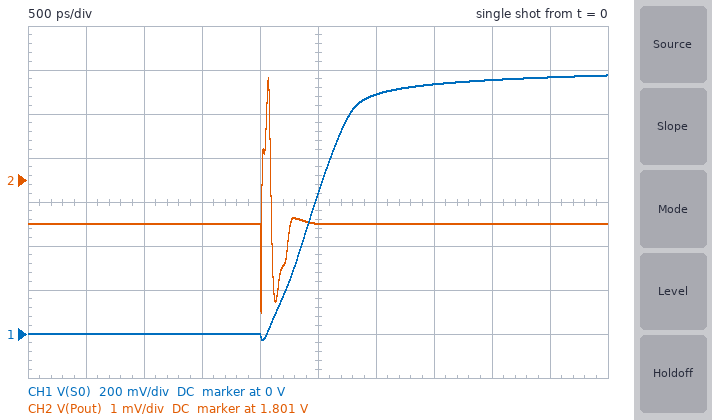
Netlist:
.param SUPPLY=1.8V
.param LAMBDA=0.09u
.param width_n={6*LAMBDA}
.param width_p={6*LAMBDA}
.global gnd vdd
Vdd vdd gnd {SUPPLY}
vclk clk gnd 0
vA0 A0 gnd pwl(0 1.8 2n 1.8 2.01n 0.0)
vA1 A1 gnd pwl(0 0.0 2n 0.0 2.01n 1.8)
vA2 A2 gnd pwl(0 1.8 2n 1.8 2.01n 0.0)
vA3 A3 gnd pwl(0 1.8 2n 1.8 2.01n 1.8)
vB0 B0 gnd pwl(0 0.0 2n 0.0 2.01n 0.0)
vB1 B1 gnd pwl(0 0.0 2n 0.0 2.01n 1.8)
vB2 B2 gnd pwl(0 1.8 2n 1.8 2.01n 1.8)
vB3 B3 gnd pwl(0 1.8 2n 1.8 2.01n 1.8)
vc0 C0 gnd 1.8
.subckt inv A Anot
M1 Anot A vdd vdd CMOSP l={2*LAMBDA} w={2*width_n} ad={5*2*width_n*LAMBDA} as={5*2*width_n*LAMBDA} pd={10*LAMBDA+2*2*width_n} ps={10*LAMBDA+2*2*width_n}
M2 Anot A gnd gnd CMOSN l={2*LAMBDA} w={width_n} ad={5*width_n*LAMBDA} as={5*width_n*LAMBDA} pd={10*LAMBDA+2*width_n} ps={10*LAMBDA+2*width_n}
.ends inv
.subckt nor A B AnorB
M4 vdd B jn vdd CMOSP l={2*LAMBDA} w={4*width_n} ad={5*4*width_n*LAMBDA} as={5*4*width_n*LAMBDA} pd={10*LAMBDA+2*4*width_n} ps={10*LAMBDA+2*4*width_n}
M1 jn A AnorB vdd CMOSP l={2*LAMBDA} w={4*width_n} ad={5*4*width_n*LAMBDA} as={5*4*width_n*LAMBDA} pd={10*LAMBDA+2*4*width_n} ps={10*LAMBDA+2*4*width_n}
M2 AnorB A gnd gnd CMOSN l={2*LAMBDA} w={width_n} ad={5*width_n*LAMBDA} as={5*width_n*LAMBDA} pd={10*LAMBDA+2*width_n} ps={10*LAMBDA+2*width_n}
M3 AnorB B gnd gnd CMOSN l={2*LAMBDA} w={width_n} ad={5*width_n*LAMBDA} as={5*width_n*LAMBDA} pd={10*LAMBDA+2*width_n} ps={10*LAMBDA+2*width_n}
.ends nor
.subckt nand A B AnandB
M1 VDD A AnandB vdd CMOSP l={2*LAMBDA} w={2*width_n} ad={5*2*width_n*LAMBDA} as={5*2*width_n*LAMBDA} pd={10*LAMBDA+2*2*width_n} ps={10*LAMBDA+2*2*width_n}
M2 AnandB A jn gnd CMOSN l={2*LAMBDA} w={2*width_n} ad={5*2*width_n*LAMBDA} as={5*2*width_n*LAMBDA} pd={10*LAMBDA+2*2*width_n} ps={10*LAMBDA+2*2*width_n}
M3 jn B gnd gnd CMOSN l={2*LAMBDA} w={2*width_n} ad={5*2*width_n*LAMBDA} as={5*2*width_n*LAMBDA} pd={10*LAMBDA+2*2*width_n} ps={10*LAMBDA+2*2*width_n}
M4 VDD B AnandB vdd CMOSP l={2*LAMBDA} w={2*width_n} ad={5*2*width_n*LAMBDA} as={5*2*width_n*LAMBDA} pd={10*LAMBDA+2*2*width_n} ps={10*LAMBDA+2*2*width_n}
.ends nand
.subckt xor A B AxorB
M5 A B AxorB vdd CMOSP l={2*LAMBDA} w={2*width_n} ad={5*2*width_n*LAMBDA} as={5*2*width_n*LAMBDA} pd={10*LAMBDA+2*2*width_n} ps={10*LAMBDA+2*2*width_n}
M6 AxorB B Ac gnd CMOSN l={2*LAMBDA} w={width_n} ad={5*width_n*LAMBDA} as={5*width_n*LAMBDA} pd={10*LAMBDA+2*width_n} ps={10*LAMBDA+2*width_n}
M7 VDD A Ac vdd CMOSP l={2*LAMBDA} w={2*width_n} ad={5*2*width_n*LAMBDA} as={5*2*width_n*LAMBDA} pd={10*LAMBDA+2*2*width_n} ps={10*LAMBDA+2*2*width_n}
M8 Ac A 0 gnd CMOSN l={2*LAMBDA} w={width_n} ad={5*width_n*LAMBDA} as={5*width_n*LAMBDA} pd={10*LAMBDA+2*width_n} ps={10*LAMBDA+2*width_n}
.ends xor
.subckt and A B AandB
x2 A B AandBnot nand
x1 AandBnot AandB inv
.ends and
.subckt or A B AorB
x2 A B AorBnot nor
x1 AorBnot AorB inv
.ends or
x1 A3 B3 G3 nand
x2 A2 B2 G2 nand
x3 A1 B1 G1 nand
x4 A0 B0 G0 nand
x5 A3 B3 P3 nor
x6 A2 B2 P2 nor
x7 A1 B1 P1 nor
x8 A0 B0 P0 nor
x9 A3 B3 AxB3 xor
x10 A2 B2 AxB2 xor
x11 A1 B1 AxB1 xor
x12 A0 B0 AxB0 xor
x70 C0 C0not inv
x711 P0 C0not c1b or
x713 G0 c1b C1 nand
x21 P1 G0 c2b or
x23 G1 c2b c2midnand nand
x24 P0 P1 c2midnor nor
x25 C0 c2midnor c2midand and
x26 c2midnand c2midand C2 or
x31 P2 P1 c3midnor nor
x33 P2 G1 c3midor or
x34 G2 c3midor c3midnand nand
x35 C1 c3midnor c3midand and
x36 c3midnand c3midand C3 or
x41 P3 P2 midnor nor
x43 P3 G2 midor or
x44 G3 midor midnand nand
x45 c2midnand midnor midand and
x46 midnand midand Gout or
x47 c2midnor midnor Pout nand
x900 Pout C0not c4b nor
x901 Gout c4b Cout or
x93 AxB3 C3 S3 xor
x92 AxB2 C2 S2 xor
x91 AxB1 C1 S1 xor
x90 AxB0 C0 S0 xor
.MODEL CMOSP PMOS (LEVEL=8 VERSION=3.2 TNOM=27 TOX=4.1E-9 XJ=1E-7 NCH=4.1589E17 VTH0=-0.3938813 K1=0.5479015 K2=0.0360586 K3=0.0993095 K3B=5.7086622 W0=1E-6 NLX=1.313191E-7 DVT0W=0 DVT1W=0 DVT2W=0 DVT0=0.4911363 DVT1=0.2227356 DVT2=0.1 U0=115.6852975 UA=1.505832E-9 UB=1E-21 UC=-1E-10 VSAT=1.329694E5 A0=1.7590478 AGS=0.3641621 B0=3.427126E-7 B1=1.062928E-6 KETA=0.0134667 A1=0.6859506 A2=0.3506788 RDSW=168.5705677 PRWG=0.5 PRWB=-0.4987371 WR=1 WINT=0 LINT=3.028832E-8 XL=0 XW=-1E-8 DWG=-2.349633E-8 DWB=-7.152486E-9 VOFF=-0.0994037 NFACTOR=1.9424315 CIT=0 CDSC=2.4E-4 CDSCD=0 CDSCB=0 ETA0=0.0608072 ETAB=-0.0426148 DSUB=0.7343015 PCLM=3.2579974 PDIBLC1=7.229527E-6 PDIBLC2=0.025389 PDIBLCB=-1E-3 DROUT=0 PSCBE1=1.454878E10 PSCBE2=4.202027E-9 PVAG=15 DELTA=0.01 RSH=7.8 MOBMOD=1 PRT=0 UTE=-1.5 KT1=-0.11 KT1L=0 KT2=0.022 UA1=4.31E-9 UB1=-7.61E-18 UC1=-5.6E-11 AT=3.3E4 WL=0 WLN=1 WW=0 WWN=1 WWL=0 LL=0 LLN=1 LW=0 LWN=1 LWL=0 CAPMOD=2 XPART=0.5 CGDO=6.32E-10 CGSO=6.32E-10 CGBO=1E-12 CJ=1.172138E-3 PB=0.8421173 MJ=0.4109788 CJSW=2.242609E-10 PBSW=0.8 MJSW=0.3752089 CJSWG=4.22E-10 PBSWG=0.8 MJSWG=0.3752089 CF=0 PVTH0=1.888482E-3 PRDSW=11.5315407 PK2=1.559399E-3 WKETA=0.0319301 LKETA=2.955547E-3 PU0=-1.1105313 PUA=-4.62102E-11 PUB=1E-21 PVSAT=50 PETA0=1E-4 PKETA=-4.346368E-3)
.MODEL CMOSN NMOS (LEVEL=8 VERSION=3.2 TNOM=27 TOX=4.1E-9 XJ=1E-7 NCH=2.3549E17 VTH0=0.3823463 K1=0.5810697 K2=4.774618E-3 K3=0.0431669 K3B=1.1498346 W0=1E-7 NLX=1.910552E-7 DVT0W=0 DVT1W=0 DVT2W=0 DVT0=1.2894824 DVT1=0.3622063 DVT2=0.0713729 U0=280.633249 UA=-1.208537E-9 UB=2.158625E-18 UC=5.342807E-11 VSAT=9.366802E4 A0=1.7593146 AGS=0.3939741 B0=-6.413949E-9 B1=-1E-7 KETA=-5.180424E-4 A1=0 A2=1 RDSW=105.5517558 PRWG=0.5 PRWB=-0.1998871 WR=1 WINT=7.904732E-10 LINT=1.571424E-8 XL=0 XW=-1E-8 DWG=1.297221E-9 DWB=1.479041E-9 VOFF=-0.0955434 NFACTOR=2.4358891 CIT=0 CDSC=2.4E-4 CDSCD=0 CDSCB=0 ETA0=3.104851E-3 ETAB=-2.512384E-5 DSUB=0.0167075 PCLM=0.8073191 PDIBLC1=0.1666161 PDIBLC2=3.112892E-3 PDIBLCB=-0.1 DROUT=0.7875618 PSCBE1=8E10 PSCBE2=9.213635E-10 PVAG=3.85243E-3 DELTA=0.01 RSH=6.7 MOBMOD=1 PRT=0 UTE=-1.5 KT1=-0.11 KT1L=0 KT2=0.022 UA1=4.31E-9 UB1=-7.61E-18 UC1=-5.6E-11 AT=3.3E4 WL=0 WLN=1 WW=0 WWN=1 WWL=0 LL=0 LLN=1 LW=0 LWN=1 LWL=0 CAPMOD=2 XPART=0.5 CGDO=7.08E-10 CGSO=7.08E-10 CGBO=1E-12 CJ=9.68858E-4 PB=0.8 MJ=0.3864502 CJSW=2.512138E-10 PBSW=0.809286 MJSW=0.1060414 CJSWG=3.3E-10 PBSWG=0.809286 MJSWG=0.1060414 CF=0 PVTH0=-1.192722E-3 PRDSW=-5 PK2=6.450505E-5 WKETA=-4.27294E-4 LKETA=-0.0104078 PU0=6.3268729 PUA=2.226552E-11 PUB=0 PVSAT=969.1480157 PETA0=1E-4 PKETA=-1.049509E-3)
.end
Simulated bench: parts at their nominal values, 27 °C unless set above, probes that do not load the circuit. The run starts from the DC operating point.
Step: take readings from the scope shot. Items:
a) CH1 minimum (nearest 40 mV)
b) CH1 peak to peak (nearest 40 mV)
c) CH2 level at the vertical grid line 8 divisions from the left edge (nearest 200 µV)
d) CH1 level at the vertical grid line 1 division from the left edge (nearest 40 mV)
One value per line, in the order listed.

-40 mV
1.20 V
1.8000 V
0 V
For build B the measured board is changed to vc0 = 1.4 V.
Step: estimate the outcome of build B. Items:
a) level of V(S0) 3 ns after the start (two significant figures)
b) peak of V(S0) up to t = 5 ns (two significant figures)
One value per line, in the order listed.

790 mV
850 mV
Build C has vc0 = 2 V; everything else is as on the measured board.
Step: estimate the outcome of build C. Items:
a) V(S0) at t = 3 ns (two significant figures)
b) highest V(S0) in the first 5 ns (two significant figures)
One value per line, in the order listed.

1.2 V
1.3 V
